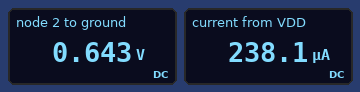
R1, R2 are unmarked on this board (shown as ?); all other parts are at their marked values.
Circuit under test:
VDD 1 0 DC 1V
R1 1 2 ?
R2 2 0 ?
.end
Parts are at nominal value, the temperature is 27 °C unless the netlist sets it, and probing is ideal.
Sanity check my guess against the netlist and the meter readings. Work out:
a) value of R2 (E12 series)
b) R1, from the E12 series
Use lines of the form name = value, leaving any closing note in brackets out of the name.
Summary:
value of R2 = 2.7 kΩ
R1, from the E12 series = 1.5 kΩ
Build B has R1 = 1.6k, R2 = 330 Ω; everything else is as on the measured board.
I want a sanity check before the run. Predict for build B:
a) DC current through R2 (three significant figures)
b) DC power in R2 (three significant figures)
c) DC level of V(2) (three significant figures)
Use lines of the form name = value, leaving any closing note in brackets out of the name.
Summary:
DC current through R2 = 518 µA
DC power in R2 = 88.6 µW
DC level of V(2) = 171 mV
